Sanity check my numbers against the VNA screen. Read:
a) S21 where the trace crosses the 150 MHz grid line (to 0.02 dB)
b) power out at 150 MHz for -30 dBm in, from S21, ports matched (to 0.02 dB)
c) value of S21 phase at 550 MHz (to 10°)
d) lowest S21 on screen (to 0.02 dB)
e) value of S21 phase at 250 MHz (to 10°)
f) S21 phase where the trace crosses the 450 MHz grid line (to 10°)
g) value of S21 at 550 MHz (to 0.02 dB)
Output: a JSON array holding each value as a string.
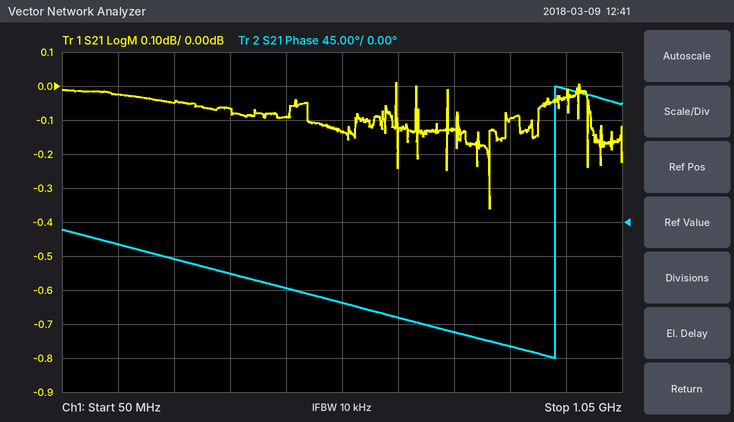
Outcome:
["-0.02 dB", "-30.02 dBm", "-110°", "-0.36 dB", "-50°", "-90°", "-0.14 dB"]
